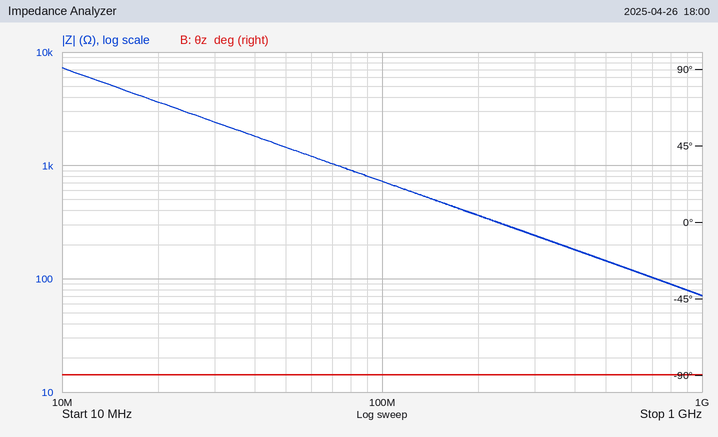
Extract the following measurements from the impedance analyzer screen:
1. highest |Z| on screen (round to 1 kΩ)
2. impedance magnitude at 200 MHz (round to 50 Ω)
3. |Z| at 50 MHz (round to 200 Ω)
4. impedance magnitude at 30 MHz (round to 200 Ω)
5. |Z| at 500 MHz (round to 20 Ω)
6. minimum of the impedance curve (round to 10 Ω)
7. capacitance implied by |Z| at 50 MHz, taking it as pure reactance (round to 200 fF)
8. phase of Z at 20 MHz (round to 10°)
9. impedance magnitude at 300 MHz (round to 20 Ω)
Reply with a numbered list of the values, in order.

1. 7 kΩ
2. 350 Ω
3. 1.4 kΩ
4. 2.4 kΩ
5. 140 Ω
6. 70 Ω
7. 2.2 pF
8. -90°
9. 240 Ω
